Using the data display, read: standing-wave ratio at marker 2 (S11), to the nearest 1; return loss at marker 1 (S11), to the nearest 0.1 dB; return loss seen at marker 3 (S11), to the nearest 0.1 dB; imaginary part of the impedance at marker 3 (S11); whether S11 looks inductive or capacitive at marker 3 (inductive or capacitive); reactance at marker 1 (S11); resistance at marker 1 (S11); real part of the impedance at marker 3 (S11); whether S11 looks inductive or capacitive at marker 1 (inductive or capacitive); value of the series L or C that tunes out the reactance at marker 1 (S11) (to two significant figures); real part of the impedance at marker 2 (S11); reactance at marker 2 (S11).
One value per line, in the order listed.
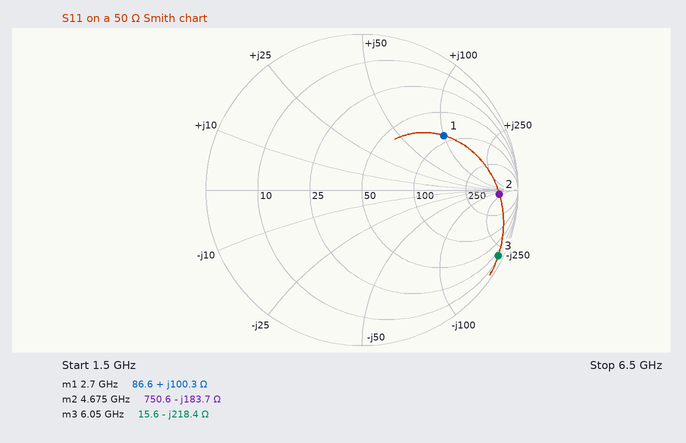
16
4.0 dB
0.3 dB
-218.4 Ω
capacitive
+100.3 Ω
86.6 Ω
15.6 Ω
inductive
590 fF
750.6 Ω
-183.7 Ω
